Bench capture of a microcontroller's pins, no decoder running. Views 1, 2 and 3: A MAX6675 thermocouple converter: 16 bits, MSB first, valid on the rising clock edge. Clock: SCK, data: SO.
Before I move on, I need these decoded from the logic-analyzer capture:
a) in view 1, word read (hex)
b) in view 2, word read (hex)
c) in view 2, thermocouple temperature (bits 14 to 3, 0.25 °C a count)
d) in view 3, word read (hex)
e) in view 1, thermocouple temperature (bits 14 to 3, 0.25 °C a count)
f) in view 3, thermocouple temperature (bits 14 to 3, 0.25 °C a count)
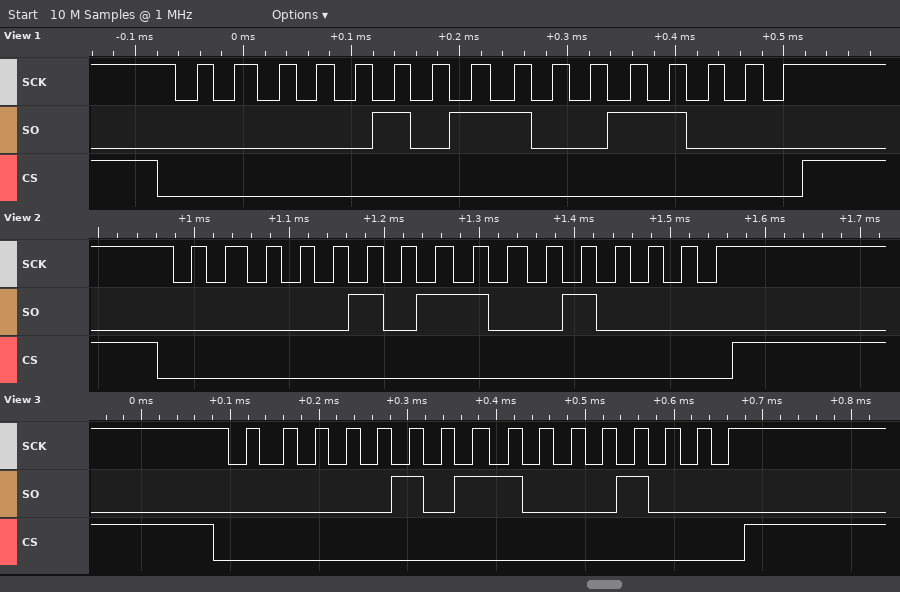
0x0598
0x0590
44.50 °C
0x0588
44.75 °C
44.25 °C
